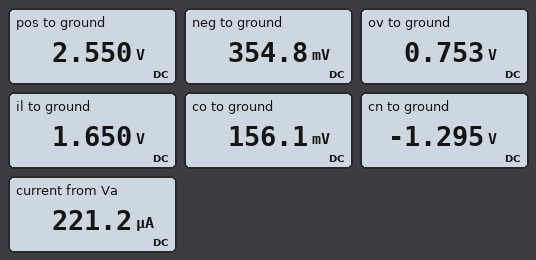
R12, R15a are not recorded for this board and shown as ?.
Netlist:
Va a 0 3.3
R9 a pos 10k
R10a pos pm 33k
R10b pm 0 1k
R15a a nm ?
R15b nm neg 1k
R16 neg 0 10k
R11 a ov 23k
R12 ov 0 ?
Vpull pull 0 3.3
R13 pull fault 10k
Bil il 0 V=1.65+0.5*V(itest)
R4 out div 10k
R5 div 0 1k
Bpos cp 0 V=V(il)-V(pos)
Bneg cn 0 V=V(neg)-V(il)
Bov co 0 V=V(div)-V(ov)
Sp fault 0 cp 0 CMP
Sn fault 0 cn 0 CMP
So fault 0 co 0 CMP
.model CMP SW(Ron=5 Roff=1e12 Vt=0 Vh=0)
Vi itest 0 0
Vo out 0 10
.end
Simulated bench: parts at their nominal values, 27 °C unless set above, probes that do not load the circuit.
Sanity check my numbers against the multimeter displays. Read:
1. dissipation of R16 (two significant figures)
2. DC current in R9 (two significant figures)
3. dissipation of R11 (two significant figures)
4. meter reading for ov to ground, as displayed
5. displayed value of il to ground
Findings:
13 µW
75 µA
280 µW
0.753 V
1.650 V
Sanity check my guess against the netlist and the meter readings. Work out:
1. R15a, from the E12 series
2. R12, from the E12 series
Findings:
82 kΩ
6.8 kΩ
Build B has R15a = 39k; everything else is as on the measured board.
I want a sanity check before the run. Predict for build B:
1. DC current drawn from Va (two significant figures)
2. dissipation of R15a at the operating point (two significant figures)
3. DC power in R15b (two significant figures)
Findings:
250 µA
170 µW
4.4 µW
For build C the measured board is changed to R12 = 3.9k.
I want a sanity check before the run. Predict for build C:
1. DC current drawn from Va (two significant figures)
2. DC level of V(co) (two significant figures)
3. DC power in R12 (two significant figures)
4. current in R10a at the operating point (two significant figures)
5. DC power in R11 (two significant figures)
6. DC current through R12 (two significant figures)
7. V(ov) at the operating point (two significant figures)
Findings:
230 µA
430 mV
59 µW
75 µA
350 µW
120 µA
480 mV
